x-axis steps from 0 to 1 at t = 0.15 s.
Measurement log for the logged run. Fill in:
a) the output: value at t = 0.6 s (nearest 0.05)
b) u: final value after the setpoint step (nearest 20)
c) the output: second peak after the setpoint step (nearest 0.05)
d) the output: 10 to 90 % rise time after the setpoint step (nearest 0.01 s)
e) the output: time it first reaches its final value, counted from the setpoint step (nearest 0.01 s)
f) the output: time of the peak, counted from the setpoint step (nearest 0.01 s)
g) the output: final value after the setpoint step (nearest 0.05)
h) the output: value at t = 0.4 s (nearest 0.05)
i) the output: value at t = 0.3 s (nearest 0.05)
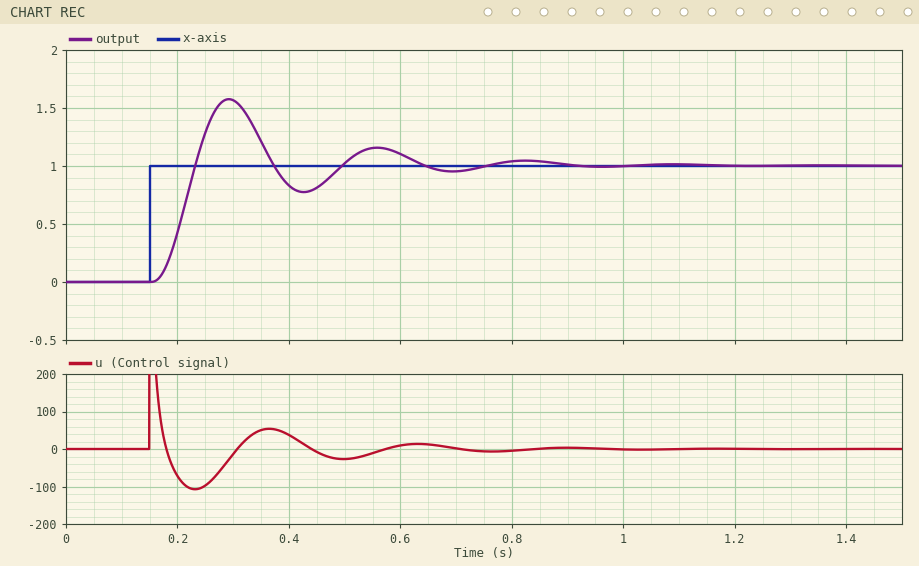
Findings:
1.10
0
1.15
0.05 s
0.08 s
0.14 s
1.00
0.85
1.55
